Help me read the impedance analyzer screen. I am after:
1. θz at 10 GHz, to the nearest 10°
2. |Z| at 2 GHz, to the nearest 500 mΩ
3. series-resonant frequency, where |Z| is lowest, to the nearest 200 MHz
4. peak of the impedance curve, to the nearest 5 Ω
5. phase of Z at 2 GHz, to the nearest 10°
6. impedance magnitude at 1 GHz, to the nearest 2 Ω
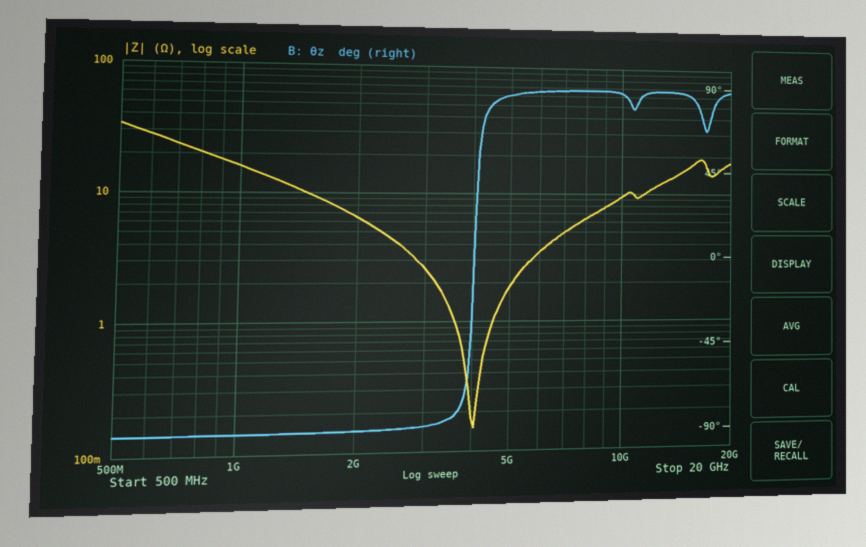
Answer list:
90°
6.5 Ω
4.0 GHz
35 Ω
-90°
16 Ω
